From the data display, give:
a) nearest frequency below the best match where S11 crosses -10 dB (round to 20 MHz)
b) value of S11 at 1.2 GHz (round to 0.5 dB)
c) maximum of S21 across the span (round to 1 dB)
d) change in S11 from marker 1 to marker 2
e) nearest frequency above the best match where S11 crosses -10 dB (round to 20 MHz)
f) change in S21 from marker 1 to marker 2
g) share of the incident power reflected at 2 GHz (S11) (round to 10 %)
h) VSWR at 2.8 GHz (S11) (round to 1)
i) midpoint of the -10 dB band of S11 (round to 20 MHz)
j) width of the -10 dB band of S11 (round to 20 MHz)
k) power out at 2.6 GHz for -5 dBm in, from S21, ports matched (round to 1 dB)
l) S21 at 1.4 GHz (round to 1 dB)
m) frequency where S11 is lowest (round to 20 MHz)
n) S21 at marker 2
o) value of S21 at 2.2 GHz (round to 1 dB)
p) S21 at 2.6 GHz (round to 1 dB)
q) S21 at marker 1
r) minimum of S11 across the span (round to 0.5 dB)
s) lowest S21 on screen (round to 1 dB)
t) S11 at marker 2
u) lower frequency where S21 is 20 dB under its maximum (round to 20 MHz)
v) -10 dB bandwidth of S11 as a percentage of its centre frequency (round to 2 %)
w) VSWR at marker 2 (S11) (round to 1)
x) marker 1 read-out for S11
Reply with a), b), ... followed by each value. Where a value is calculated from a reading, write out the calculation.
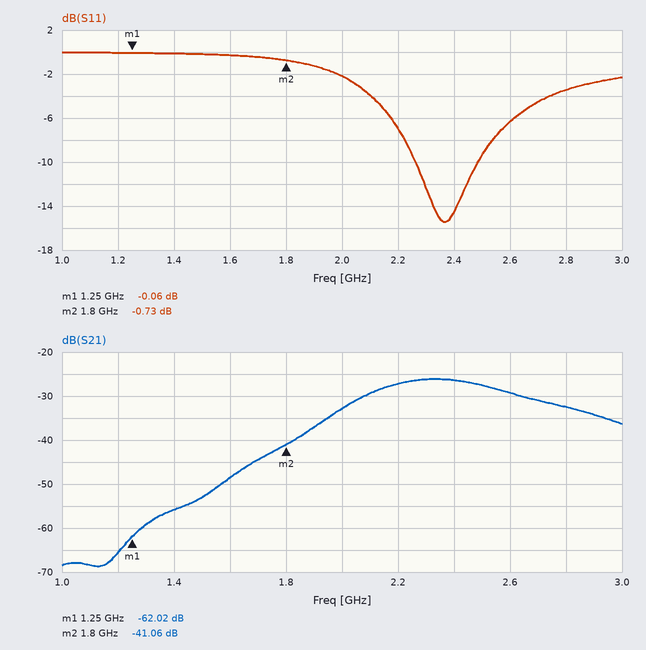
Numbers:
a) 2.26 GHz
b) 0.0 dB
c) -26 dB
d) -0.73 − (-0.06) = -0.67 dB
e) 2.48 GHz
f) -41.06 − (-62.02) = 20.96 dB
g) 10^(-2/10) ≈ 63.1 %, so 60 % to the nearest 10 %
h) |Γ| = 10^(-3.5/20) = 0.6683; VSWR = (1 + 0.6683)/(1 − 0.6683) ≈ 5
i) 2.38 GHz
j) 2.48 GHz − 2.26 GHz = 220 MHz
k) -5 dBm + (-29 dB) = -34 dBm
l) -56 dB
m) 2.36 GHz
n) -41.06 dB
o) -27 dB
p) -29 dB
q) -62.02 dB
r) -15.5 dB
s) -69 dB
t) -0.73 dB
u) 1.66 GHz
v) 220 MHz / 2.37 GHz ≈ 9.28 %, so 10 % to the nearest 2 %
w) (1 + 0.9194)/(1 − 0.9194) ≈ 24
x) -0.06 dB
